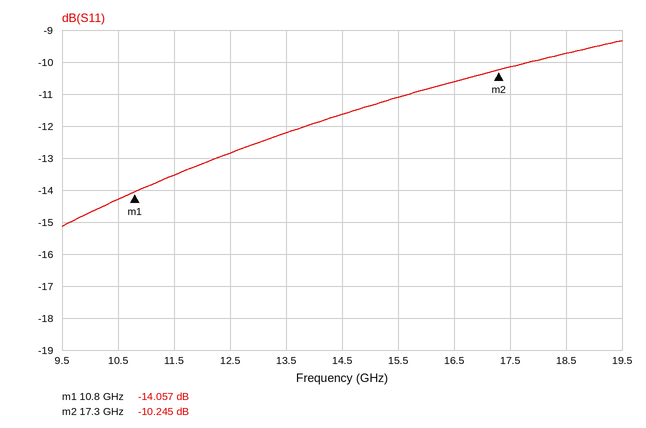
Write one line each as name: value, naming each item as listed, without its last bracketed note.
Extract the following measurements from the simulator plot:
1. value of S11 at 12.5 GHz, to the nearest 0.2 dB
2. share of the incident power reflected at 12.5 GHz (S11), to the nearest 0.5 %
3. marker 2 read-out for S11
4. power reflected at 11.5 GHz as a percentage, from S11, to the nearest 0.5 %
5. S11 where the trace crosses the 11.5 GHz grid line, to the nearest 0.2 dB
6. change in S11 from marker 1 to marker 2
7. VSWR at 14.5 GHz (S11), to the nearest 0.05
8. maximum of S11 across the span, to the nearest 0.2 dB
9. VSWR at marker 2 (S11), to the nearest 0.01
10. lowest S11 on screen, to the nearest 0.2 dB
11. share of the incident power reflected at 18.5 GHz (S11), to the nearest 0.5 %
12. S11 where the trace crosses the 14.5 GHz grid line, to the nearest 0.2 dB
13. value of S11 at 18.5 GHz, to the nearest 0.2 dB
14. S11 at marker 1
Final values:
value of S11 at 12.5 GHz, to the nearest 0.2 dB: -12.8 dB
share of the incident power reflected at 12.5 GHz (S11), to the nearest 0.5 %: 5.0 %
marker 2 read-out for S11: -10.245 dB
power reflected at 11.5 GHz as a percentage, from S11, to the nearest 0.5 %: 4.5 %
S11 where the trace crosses the 11.5 GHz grid line, to the nearest 0.2 dB: -13.6 dB
change in S11 from marker 1 to marker 2: 3.812 dB
VSWR at 14.5 GHz (S11), to the nearest 0.05: 1.70
maximum of S11 across the span, to the nearest 0.2 dB: -9.4 dB
VSWR at marker 2 (S11), to the nearest 0.01: 1.89
lowest S11 on screen, to the nearest 0.2 dB: -15.2 dB
share of the incident power reflected at 18.5 GHz (S11), to the nearest 0.5 %: 10.5 %
S11 where the trace crosses the 14.5 GHz grid line, to the nearest 0.2 dB: -11.6 dB
value of S11 at 18.5 GHz, to the nearest 0.2 dB: -9.8 dB
S11 at marker 1: -14.057 dB
